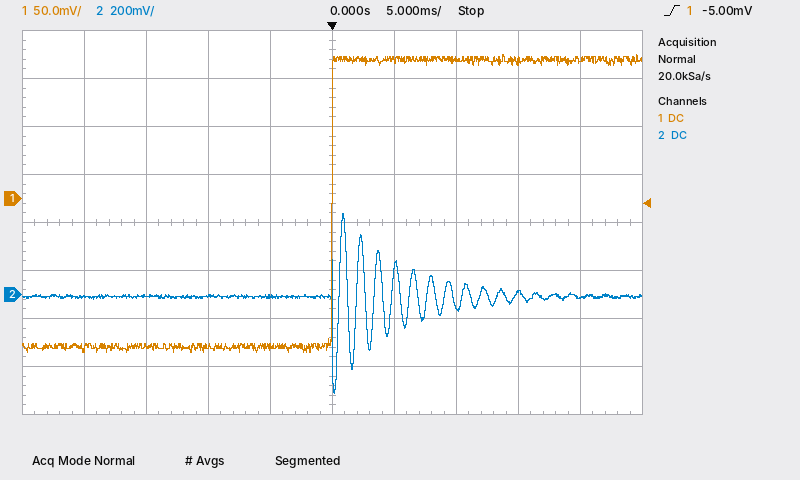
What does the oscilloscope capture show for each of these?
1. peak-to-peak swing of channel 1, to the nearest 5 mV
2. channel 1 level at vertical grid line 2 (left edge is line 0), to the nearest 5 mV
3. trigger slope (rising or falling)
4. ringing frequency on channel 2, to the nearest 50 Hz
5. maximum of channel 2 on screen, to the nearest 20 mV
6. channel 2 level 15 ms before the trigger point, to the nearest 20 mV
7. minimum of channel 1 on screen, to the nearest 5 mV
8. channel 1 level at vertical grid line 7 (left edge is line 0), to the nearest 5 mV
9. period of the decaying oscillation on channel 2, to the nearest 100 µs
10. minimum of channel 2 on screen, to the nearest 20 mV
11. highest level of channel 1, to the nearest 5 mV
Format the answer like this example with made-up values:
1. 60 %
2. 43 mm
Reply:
1. 310 mV
2. -155 mV
3. rising
4. 700 Hz
5. 340 mV
6. 0 mV
7. -160 mV
8. 145 mV
9. 1.4 ms
10. -420 mV
11. 150 mV
